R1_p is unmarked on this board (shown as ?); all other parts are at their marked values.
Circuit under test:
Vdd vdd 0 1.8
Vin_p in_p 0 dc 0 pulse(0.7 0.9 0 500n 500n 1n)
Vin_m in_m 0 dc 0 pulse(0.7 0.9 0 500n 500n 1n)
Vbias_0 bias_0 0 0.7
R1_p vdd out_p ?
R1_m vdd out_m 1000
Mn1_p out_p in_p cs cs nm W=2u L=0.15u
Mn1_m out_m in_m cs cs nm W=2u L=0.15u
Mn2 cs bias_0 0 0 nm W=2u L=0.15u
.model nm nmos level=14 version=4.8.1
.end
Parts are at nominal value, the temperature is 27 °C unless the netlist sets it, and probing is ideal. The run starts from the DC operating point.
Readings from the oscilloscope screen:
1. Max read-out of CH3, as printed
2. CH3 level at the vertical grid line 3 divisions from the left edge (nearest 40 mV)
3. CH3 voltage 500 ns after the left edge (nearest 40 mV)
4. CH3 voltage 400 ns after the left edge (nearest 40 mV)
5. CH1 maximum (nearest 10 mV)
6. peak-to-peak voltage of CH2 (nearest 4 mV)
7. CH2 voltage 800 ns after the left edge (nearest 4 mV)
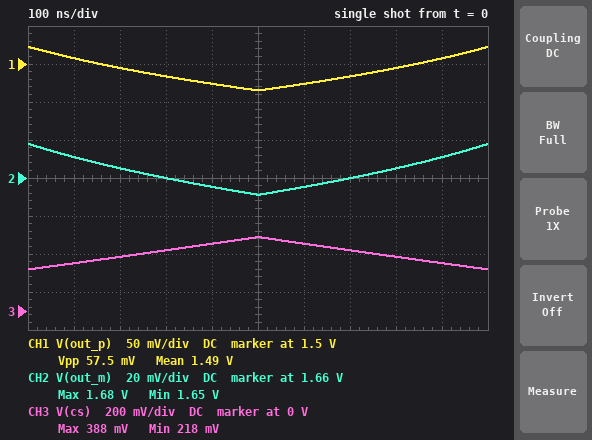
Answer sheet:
388 mV
320 mV
400 mV
360 mV
1.52 V
28 mV
1.664 V
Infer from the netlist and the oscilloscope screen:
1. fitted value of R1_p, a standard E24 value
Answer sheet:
2.4 kΩ
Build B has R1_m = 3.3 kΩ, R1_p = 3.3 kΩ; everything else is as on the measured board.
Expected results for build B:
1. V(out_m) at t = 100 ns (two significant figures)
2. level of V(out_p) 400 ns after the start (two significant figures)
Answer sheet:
1.4 V
1.3 V
